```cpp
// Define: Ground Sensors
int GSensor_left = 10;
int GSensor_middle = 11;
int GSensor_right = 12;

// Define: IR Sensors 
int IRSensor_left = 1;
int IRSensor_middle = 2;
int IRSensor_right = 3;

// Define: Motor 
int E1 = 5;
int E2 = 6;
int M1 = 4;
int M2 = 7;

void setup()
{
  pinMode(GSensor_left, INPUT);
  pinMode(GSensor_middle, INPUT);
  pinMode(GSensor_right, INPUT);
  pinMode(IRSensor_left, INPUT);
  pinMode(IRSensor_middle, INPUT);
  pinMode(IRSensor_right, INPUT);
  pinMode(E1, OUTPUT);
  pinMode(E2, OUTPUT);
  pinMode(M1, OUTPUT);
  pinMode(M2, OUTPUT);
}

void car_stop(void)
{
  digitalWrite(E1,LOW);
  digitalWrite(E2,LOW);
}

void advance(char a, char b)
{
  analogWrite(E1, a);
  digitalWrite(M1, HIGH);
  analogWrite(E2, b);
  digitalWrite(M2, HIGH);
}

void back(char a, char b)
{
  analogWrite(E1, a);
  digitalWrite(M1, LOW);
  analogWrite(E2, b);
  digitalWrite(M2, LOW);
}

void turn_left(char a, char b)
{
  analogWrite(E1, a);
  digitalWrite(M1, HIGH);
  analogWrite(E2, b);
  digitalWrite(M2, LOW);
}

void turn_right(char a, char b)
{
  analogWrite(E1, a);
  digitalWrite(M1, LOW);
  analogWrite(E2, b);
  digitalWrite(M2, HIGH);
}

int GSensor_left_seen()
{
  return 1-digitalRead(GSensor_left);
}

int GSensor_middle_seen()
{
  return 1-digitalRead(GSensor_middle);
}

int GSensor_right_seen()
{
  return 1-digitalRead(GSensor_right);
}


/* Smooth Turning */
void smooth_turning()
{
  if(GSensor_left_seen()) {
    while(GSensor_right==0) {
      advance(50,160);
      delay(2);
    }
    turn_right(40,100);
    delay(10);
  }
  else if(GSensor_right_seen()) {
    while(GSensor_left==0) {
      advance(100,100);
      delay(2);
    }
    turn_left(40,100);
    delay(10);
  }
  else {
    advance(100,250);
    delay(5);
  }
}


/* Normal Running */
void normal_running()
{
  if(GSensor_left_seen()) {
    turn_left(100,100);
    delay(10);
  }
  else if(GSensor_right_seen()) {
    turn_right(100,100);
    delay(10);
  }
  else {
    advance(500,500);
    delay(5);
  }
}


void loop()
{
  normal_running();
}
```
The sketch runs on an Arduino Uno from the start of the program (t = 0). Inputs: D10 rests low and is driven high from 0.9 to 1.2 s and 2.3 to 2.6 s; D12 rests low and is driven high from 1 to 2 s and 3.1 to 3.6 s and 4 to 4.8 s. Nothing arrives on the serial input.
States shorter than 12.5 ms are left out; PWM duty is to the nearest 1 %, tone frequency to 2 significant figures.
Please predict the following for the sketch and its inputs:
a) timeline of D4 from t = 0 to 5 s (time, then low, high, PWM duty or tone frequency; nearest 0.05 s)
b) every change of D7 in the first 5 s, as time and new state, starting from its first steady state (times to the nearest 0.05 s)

0 s high; 0.9 s low; 1 s high; 2.3 s low; 2.6 s high
0 s low; 0.9 s high; 1.2 s low; 2.3 s high; 2.6 s low
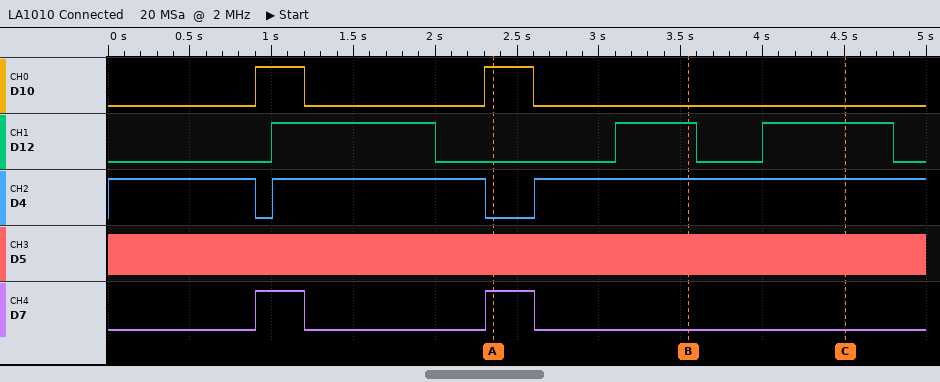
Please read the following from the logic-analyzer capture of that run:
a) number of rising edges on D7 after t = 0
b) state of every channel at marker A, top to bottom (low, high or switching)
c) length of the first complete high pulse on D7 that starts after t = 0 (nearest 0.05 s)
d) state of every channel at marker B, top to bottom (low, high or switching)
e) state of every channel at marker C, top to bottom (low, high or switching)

2
D10 high, D12 low, D4 low, D5 switching, D7 high
0.30 s
D10 low, D12 high, D4 high, D5 switching, D7 low
D10 low, D12 high, D4 high, D5 switching, D7 low
